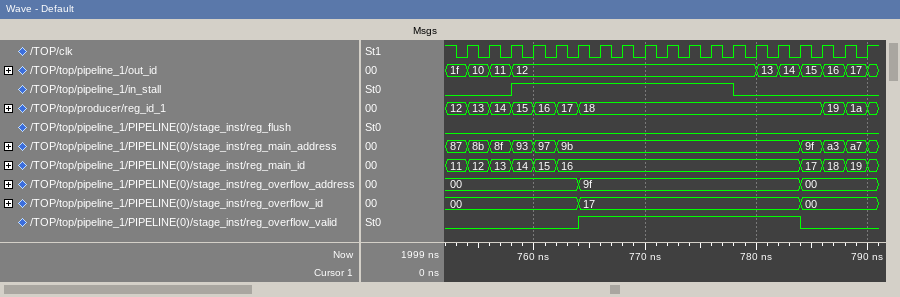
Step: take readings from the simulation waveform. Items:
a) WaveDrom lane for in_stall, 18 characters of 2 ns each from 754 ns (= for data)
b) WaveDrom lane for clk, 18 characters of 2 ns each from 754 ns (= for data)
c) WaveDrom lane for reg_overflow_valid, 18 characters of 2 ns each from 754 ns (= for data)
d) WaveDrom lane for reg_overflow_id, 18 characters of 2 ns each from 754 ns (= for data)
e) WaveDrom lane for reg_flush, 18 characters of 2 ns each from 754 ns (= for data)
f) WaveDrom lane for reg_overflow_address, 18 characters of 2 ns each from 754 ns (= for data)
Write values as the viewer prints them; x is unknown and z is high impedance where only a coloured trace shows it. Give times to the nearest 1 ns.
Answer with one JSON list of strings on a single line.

["{name: 'in_stall', wave: '0.1.........0.....'}", "{name: 'clk', wave: 'p.................'}", "{name: 'reg_overflow_valid', wave: '0....1.........0..'}", "{name: 'reg_overflow_id', wave: '=....=.........=..', data: '00 17 00'}", "{name: 'reg_flush', wave: '0.................'}", "{name: 'reg_overflow_address', wave: '=....=.........=..', data: '00 9f 00'}"]
